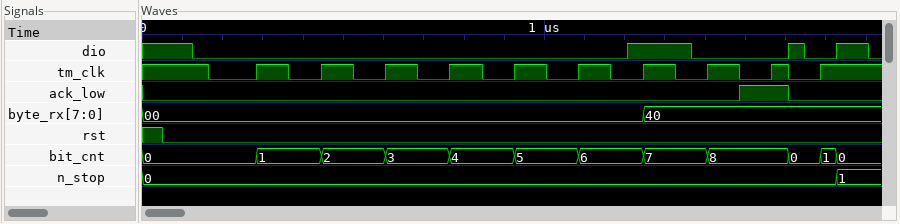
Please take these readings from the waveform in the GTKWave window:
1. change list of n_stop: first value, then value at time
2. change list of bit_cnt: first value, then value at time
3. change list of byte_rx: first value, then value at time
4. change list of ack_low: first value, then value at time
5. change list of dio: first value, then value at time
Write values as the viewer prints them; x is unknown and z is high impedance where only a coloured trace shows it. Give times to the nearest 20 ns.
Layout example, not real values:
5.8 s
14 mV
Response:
0, 1 at 1720 ns
0, 1 at 280 ns, 2 at 440 ns, 3 at 600 ns, 4 at 760 ns, 5 at 920 ns, 6 at 1080 ns, 7 at 1240 ns, 8 at 1400 ns, 0 at 1600 ns, 1 at 1680 ns, 0 at 1720 ns
00, 40 at 1240 ns
0, 1 at 1480 ns, 0 at 1600 ns
1, 0 at 120 ns, 1 at 1200 ns, 0 at 1360 ns, 1 at 1600 ns, 0 at 1640 ns, 1 at 1720 ns, 0 at 1800 ns
